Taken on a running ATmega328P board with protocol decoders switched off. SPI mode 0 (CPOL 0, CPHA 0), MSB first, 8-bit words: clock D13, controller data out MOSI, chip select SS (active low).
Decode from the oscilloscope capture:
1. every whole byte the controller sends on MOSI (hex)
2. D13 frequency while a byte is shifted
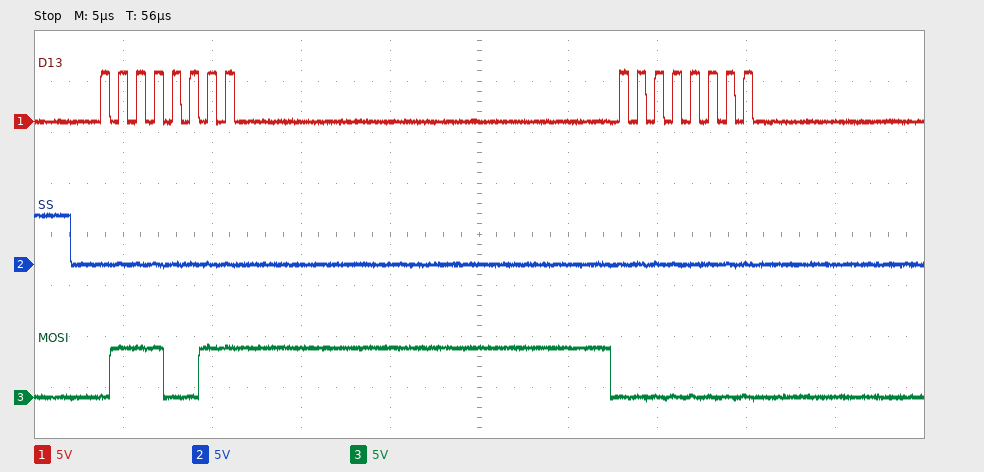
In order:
73 00
1 MHz
